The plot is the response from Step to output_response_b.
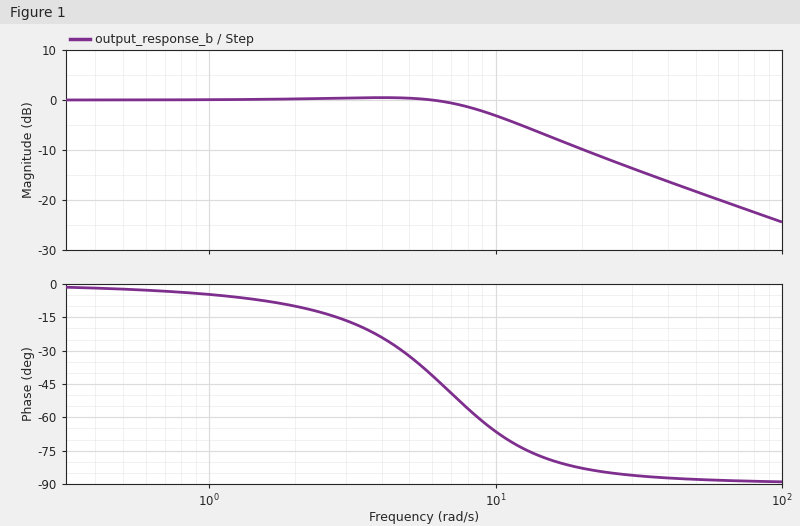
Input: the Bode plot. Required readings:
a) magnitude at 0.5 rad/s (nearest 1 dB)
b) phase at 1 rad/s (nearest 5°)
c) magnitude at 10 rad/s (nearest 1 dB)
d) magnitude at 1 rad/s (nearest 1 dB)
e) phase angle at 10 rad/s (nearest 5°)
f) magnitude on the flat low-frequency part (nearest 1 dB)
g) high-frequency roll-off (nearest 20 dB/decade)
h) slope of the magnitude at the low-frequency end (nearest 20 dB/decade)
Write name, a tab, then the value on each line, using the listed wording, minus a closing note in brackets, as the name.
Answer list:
magnitude at 0.5 rad/s	0 dB
phase at 1 rad/s	-5°
magnitude at 10 rad/s	-3 dB
magnitude at 1 rad/s	0 dB
phase angle at 10 rad/s	-65°
magnitude on the flat low-frequency part	0 dB
high-frequency roll-off	-20 dB/decade
slope of the magnitude at the low-frequency end	0 dB/decade
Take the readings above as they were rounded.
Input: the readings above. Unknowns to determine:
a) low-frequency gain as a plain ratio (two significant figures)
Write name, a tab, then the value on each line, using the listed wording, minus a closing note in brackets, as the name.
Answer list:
low-frequency gain as a plain ratio	1.0
